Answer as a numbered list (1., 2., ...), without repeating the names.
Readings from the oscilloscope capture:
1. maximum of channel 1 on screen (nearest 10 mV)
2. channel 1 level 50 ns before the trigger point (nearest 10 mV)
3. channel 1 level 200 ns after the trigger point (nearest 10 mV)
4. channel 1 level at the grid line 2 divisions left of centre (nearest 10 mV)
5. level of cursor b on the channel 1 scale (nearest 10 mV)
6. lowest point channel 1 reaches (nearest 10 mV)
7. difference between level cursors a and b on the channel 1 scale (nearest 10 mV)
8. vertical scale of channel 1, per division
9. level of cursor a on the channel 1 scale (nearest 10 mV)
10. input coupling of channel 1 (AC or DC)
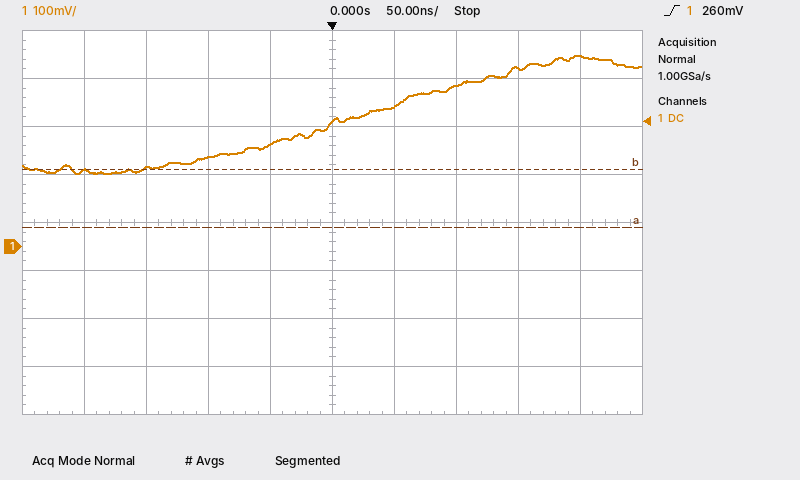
1. 400 mV
2. 210 mV
3. 400 mV
4. 190 mV
5. 160 mV
6. 150 mV
7. 120 mV
8. 100 mV
9. 40 mV
10. DC
